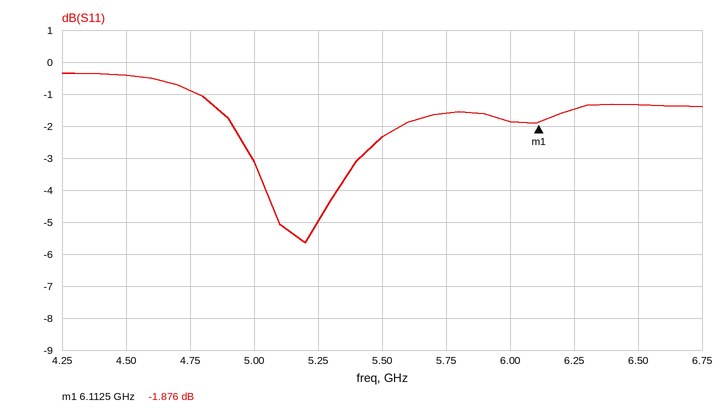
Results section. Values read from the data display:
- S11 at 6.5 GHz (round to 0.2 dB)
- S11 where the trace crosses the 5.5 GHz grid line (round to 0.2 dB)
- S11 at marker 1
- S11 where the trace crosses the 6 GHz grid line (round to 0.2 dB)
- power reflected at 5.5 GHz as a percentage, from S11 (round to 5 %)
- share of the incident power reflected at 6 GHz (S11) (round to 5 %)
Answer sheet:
-1.4 dB
-2.4 dB
-1.876 dB
-1.8 dB
60 %
65 %
